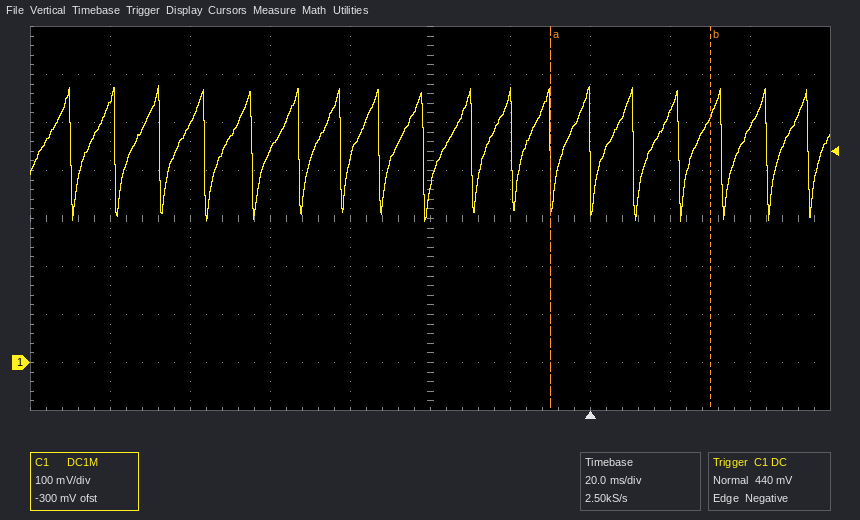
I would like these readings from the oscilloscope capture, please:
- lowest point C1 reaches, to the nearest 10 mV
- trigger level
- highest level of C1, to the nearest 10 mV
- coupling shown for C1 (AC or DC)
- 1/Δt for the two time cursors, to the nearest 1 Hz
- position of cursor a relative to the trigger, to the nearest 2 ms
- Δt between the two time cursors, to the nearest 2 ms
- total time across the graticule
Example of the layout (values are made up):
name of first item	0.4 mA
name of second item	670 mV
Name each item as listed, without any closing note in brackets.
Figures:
lowest point C1 reaches, to the nearest 10 mV	290 mV
trigger level	440 mV
highest level of C1, to the nearest 10 mV	580 mV
coupling shown for C1	DC
1/Δt for the two time cursors, to the nearest 1 Hz	25 Hz
position of cursor a relative to the trigger, to the nearest 2 ms	-10 ms
Δt between the two time cursors, to the nearest 2 ms	40 ms
total time across the graticule	200 ms
